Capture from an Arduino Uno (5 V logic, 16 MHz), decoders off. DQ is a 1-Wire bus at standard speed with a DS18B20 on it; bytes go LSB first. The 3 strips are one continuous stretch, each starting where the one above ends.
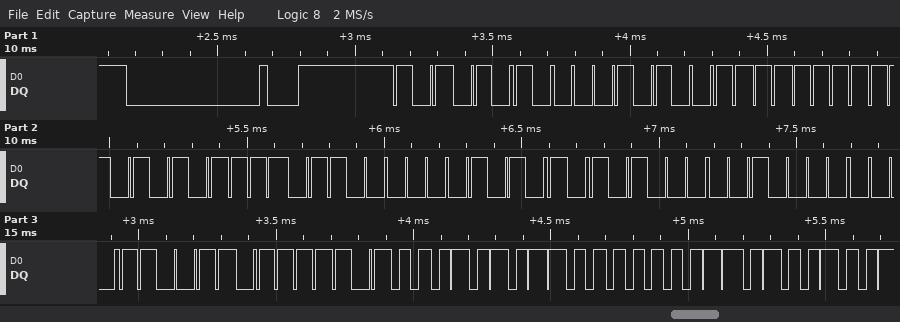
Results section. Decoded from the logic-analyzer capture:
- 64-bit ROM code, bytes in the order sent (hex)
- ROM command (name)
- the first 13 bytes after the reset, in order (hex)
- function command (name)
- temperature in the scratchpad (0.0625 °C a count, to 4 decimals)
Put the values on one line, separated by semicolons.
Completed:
28 FF AB 37 50 15 04 CC; Match ROM; 55 28 FF AB 37 50 15 04 CC BE A8 01 4B; Read Scratchpad; 26.5000 °C
